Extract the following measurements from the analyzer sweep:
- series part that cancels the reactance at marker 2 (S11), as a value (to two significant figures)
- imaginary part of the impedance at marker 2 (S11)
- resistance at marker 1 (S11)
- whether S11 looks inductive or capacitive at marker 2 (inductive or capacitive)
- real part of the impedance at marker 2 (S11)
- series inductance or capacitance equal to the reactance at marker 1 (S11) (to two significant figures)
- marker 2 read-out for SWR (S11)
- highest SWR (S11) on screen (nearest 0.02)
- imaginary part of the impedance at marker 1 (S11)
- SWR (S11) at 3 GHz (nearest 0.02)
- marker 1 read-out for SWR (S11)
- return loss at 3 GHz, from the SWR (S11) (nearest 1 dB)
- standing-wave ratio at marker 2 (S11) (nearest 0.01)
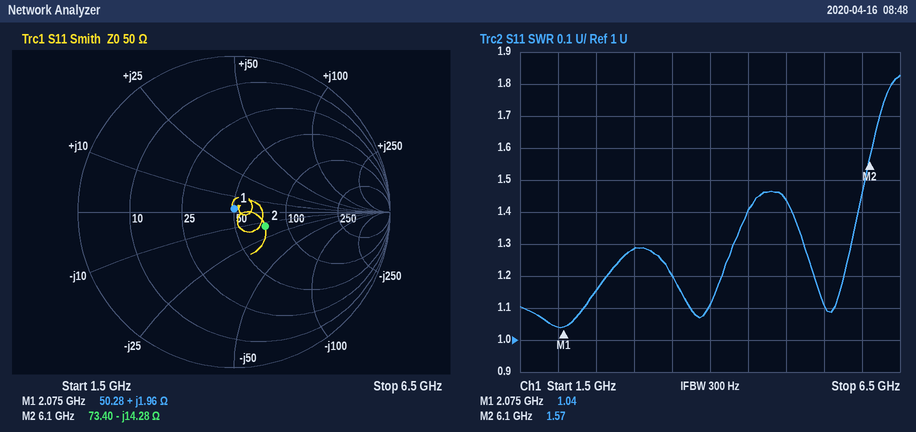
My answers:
370 pH
-14.28 Ω
50.28 Ω
capacitive
73.40 Ω
150 pH
1.57
1.82
+1.96 Ω
1.28
1.04
18 dB
1.57
